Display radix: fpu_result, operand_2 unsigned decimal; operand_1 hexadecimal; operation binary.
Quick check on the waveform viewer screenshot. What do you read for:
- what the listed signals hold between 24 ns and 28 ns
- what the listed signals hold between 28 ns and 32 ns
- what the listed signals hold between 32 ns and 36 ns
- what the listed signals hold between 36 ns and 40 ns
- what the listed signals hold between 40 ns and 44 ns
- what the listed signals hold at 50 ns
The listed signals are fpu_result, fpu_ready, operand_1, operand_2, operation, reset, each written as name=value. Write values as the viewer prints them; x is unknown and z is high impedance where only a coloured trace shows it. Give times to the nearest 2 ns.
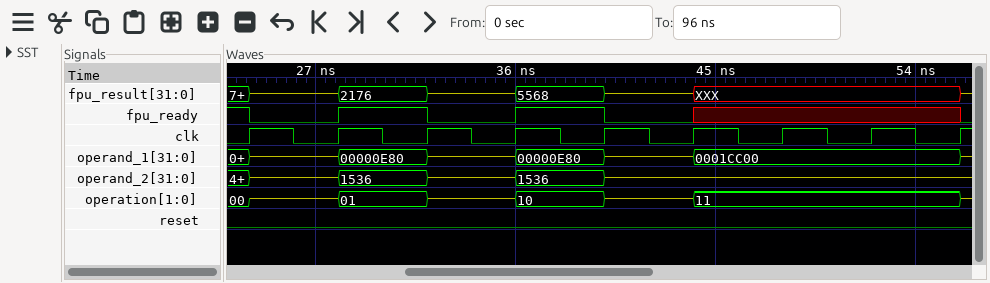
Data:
fpu_result=z, fpu_ready=0, operand_1=z, operand_2=z, operation=z, reset=0
fpu_result=2176, fpu_ready=1, operand_1=00000E80, operand_2=1536, operation=01, reset=0
fpu_result=z, fpu_ready=0, operand_1=z, operand_2=z, operation=z, reset=0
fpu_result=5568, fpu_ready=1, operand_1=00000E80, operand_2=1536, operation=10, reset=0
fpu_result=z, fpu_ready=0, operand_1=z, operand_2=z, operation=z, reset=0
fpu_result=XXX, fpu_ready=x, operand_1=0001CC00, operand_2=z, operation=11, reset=0
